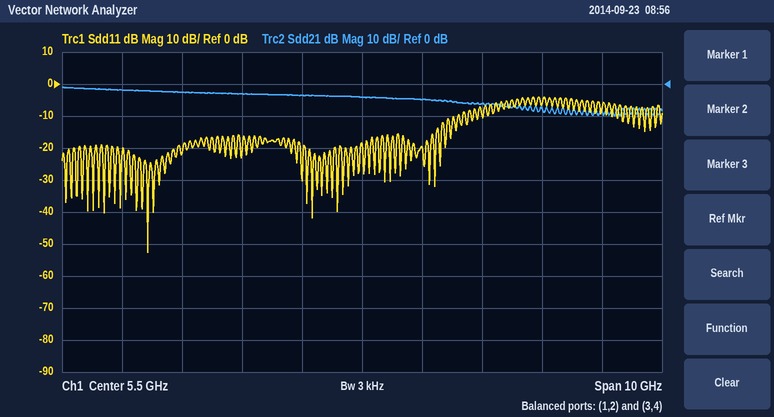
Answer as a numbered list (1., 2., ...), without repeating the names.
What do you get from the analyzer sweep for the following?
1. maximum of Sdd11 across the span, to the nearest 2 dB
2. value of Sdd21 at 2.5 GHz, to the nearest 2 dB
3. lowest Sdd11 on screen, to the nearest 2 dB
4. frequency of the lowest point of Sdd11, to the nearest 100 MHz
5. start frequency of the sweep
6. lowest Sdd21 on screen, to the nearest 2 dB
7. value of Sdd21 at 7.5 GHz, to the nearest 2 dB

1. -4 dB
2. -2 dB
3. -52 dB
4. 1.9 GHz
5. 500 MHz
6. -10 dB
7. -6 dB
